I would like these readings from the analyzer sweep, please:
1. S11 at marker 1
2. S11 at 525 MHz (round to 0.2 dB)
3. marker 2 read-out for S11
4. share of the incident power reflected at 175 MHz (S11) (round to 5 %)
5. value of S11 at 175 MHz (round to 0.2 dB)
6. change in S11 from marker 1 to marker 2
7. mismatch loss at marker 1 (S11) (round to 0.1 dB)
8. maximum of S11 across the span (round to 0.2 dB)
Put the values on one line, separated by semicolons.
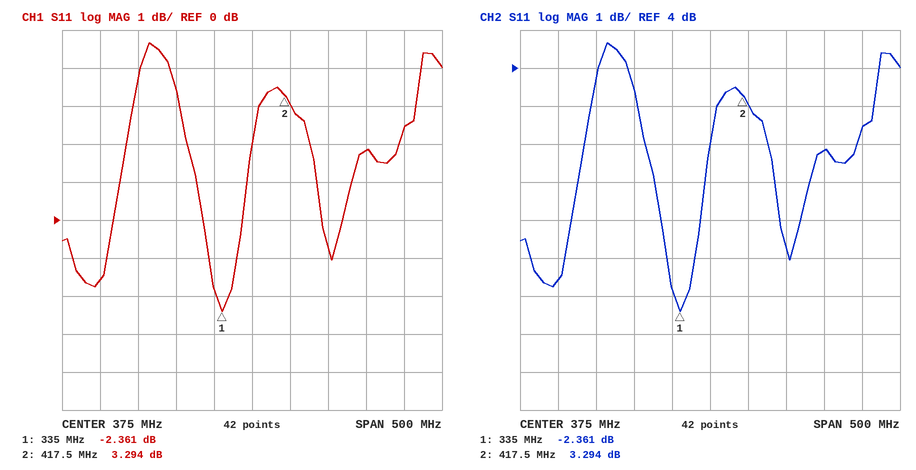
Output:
-2.361 dB; 1.8 dB; 3.294 dB; 70 %; -1.6 dB; 5.655 dB; 3.8 dB; 4.6 dB
